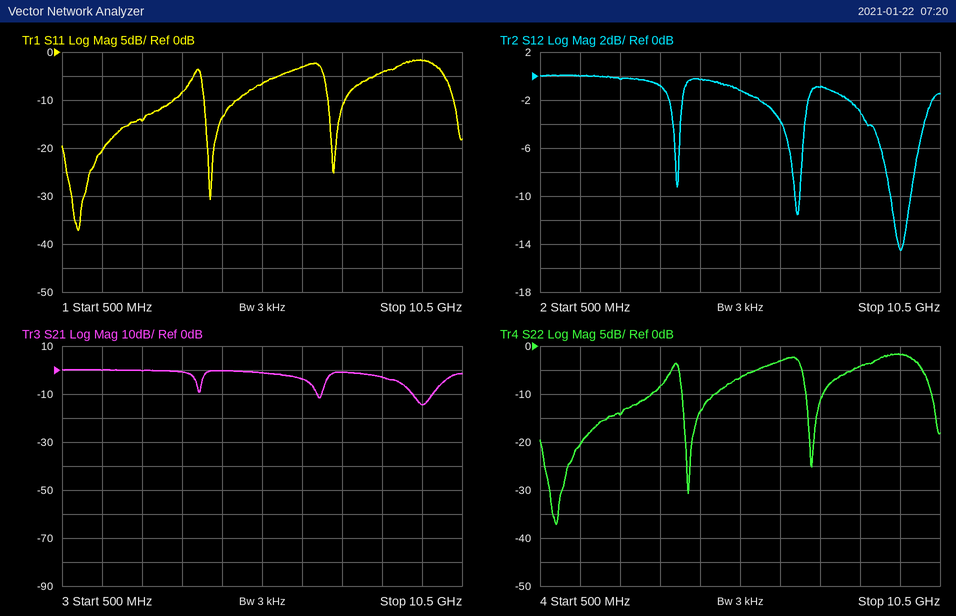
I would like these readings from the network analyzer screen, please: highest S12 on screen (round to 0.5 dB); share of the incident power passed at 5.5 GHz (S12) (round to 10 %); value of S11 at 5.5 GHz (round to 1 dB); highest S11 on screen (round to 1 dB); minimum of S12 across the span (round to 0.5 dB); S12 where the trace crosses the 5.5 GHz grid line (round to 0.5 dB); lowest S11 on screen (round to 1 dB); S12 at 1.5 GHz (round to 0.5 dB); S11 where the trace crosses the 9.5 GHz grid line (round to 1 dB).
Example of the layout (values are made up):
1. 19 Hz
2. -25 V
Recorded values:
1. 0.0 dB
2. 80 %
3. -7 dB
4. -2 dB
5. -14.5 dB
6. -1.0 dB
7. -37 dB
8. 0.0 dB
9. -2 dB
